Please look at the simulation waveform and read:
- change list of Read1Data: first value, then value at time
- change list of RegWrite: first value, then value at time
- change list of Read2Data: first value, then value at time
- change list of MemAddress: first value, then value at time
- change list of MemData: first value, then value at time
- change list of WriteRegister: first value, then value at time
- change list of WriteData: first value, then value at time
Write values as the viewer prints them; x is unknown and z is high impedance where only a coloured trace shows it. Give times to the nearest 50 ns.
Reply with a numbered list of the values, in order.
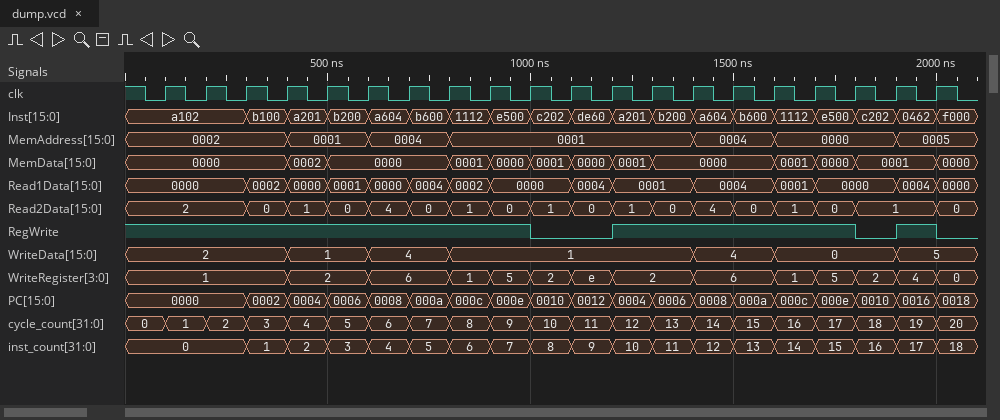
1. 0000, 0002 at 300 ns, 0000 at 400 ns, 0001 at 500 ns, 0000 at 600 ns, 0004 at 700 ns, 0002 at 800 ns, 0000 at 900 ns, 0004 at 1100 ns, 0001 at 1200 ns, 0004 at 1400 ns, 0001 at 1600 ns, 0000 at 1700 ns, 0004 at 1900 ns, 0000 at 2000 ns
2. 1, 0 at 1000 ns, 1 at 1200 ns, 0 at 1800 ns, 1 at 1900 ns, 0 at 2000 ns
3. 2, 0 at 300 ns, 1 at 400 ns, 0 at 500 ns, 4 at 600 ns, 0 at 700 ns, 1 at 800 ns, 0 at 900 ns, 1 at 1000 ns, 0 at 1100 ns, 1 at 1200 ns, 0 at 1300 ns, 4 at 1400 ns, 0 at 1500 ns, 1 at 1600 ns, 0 at 1700 ns, 1 at 1800 ns, 0 at 2000 ns
4. 0002, 0001 at 400 ns, 0004 at 600 ns, 0001 at 800 ns, 0004 at 1400 ns, 0000 at 1600 ns, 0005 at 1900 ns
5. 0000, 0002 at 400 ns, 0000 at 500 ns, 0001 at 800 ns, 0000 at 900 ns, 0001 at 1000 ns, 0000 at 1100 ns, 0001 at 1200 ns, 0000 at 1300 ns, 0001 at 1600 ns, 0000 at 1700 ns, 0001 at 1800 ns, 0000 at 2000 ns
6. 1, 2 at 400 ns, 6 at 600 ns, 1 at 800 ns, 5 at 900 ns, 2 at 1000 ns, e at 1100 ns, 2 at 1200 ns, 6 at 1400 ns, 1 at 1600 ns, 5 at 1700 ns, 2 at 1800 ns, 4 at 1900 ns, 0 at 2000 ns
7. 2, 1 at 400 ns, 4 at 600 ns, 1 at 800 ns, 4 at 1400 ns, 0 at 1600 ns, 5 at 1900 ns
